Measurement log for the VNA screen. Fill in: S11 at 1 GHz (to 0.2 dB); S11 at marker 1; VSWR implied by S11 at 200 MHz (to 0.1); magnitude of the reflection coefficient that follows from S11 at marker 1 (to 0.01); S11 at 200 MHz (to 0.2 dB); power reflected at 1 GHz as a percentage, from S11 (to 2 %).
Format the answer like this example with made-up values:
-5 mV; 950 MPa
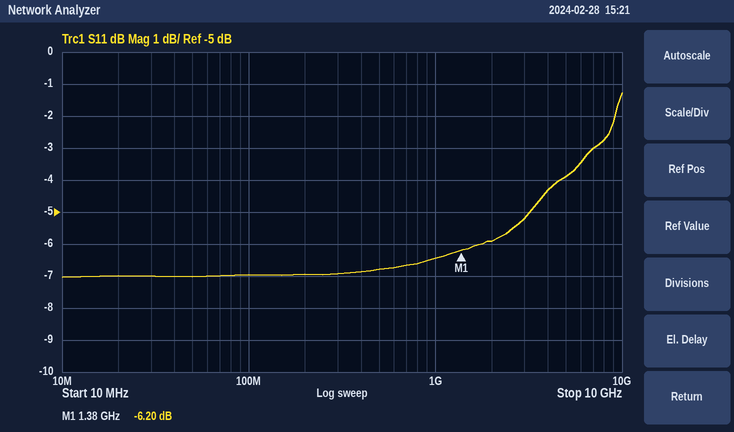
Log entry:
-6.4 dB; -6.20 dB; 2.6; 0.49; -7.0 dB; 22 %
